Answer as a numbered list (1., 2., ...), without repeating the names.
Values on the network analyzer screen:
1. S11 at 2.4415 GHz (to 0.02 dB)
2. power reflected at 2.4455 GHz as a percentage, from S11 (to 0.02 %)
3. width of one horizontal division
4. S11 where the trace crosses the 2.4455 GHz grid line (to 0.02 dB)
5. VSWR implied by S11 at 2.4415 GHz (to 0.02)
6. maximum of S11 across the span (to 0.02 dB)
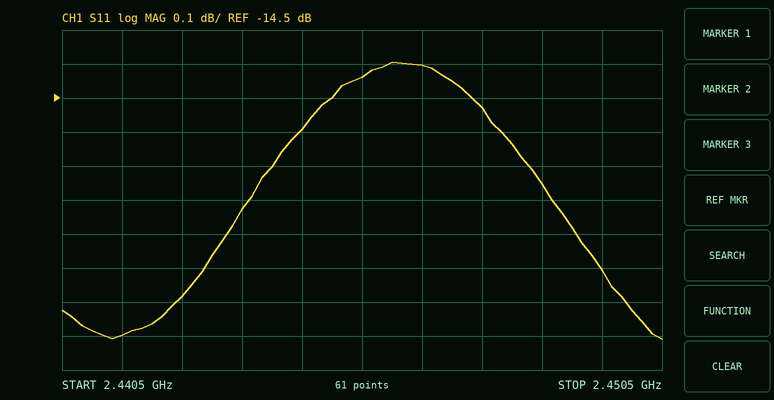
1. -15.20 dB
2. 3.60 %
3. 1 MHz
4. -14.44 dB
5. 1.42
6. -14.40 dB
